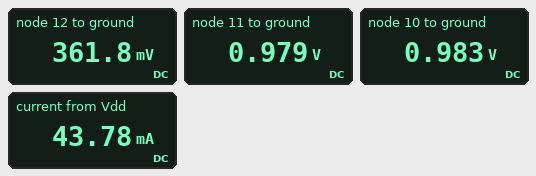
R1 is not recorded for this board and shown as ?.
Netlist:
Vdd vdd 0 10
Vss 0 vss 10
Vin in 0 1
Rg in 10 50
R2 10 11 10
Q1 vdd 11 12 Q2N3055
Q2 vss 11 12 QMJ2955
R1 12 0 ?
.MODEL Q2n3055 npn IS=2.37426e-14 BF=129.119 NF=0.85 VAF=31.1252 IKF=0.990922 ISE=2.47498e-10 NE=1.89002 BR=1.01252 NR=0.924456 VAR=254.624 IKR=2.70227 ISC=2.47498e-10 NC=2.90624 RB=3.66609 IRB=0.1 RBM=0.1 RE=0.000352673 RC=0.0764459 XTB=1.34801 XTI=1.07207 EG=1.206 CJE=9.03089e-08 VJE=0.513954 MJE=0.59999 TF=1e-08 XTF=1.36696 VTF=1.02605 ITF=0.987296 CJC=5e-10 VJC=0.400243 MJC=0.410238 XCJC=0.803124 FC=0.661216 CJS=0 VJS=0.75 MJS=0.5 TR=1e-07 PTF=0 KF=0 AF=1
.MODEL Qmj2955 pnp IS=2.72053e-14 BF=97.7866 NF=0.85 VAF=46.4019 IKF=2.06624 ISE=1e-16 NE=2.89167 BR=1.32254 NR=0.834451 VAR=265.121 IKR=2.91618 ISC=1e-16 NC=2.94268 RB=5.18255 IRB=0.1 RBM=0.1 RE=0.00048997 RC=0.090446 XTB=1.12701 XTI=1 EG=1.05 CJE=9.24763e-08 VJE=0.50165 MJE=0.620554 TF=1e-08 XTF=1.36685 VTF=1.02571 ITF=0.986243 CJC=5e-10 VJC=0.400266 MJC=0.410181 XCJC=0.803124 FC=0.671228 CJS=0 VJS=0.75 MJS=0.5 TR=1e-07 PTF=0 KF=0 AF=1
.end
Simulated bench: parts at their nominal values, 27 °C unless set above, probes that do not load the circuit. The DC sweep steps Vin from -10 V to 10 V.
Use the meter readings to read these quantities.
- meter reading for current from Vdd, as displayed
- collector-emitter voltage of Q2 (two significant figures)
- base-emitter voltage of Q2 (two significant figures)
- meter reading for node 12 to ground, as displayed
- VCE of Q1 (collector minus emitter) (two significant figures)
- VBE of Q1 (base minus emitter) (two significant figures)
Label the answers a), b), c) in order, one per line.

a) 43.78 mA
b) -10 V
c) 620 mV
d) 361.8 mV
e) 9.6 V
f) 620 mV
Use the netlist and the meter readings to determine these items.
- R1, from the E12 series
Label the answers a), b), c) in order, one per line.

a) 8.2 Ω
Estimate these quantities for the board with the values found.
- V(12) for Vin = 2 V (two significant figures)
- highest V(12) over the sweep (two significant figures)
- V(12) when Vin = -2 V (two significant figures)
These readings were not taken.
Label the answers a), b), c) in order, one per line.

a) 1.3 V
b) 8.3 V
c) -1.3 V
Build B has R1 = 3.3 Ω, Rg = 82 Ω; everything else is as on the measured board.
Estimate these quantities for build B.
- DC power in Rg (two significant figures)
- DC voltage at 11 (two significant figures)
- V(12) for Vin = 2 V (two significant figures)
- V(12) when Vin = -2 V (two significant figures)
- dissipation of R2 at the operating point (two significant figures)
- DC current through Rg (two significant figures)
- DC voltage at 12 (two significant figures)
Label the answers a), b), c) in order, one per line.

a) 39 µW
b) 940 mV
c) 1.1 V
d) -1.0 V
e) 4.7 µW
f) 690 µA
g) 300 mV
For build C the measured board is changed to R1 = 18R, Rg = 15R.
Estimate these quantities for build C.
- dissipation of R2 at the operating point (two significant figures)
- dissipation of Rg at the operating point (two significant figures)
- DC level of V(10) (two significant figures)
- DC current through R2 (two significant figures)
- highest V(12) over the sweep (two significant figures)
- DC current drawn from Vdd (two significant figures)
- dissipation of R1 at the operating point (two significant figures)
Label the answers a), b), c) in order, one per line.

a) 350 nW
b) 520 nW
c) 1.0 V
d) 190 µA
e) 9.1 V
f) 22 mA
g) 8.6 mW
